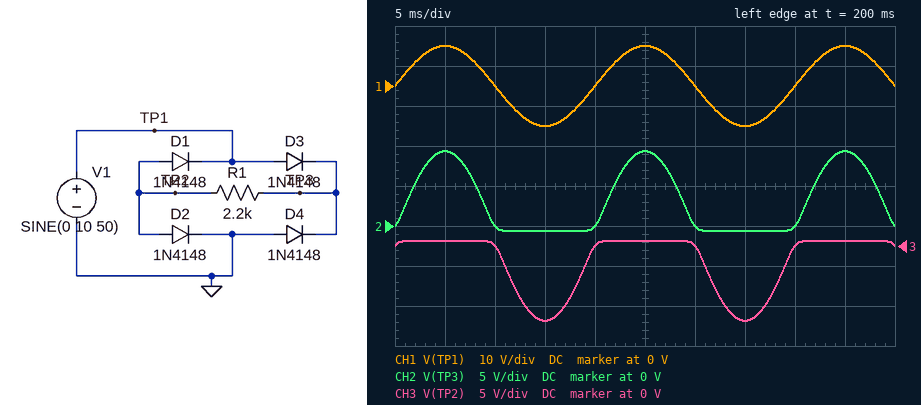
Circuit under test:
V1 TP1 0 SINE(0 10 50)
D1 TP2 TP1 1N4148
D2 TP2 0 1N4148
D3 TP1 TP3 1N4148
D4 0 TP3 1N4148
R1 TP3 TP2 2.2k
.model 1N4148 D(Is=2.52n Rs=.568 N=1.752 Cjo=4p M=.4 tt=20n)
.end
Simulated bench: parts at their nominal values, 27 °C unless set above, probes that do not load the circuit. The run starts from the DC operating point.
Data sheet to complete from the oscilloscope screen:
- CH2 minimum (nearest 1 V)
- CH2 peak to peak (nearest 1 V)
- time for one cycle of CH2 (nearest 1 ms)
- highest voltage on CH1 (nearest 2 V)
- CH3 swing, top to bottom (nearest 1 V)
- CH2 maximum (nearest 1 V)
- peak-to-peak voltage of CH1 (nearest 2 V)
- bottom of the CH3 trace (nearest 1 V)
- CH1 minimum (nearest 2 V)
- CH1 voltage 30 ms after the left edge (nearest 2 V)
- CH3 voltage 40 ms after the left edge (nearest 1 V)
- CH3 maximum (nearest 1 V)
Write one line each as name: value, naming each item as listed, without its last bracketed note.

CH2 minimum: -1 V
CH2 peak to peak: 10 V
time for one cycle of CH2: 20 ms
highest voltage on CH1: 10 V
CH3 swing, top to bottom: 10 V
CH2 maximum: 9 V
peak-to-peak voltage of CH1: 20 V
bottom of the CH3 trace: -9 V
CH1 minimum: -10 V
CH1 voltage 30 ms after the left edge: 0 V
CH3 voltage 40 ms after the left edge: 0 V
CH3 maximum: 1 V
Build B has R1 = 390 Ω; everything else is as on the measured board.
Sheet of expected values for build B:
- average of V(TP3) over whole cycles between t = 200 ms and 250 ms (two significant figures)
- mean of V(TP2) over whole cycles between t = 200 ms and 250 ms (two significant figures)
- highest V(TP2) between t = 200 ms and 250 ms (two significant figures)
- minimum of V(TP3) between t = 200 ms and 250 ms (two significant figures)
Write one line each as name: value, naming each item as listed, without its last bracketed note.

average of V(TP3) over whole cycles between t = 200 ms and 250 ms: 2.5 V
mean of V(TP2) over whole cycles between t = 200 ms and 250 ms: -2.5 V
highest V(TP2) between t = 200 ms and 250 ms: 740 mV
minimum of V(TP3) between t = 200 ms and 250 ms: -740 mV
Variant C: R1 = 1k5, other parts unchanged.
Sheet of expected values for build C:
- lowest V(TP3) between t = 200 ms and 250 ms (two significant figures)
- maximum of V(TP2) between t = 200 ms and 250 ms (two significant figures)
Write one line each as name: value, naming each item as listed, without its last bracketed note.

lowest V(TP3) between t = 200 ms and 250 ms: -670 mV
maximum of V(TP2) between t = 200 ms and 250 ms: 670 mV
